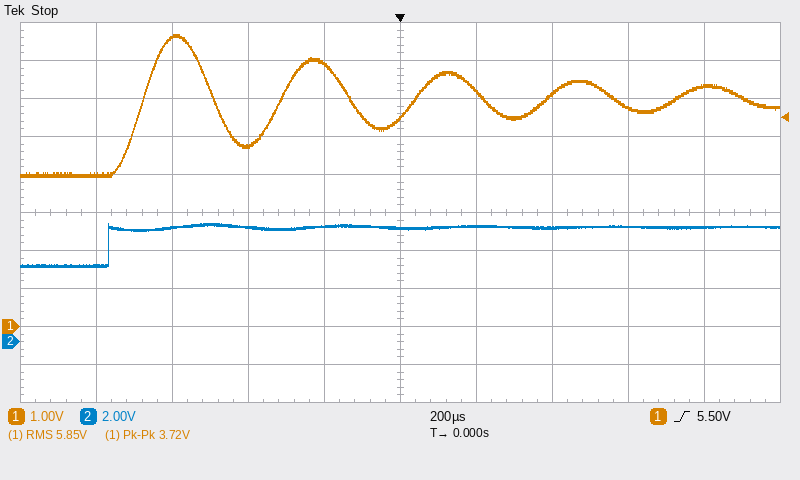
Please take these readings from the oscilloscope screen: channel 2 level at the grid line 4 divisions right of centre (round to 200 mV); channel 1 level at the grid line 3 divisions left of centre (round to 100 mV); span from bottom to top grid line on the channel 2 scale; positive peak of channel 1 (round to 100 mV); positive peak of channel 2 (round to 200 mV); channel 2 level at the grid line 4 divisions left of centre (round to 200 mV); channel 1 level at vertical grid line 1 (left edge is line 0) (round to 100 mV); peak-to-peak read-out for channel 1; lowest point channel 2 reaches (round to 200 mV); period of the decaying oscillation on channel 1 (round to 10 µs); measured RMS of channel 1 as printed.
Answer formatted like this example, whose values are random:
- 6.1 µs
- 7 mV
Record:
- 6.0 V
- 7.6 V
- 20 V
- 7.7 V
- 6.2 V
- 4.0 V
- 4.0 V
- 3.72 V
- 4.0 V
- 350 µs
- 5.85 V
